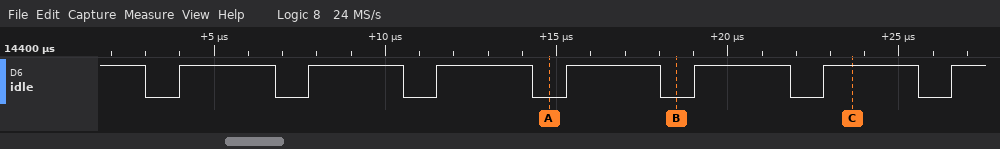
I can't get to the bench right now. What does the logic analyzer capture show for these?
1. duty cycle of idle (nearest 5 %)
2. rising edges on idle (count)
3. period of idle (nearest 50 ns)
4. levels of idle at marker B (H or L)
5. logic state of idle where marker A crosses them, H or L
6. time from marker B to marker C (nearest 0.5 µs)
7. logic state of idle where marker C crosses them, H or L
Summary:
75 %
7
3750 ns
idle=L
idle=L
5 µs
idle=H
